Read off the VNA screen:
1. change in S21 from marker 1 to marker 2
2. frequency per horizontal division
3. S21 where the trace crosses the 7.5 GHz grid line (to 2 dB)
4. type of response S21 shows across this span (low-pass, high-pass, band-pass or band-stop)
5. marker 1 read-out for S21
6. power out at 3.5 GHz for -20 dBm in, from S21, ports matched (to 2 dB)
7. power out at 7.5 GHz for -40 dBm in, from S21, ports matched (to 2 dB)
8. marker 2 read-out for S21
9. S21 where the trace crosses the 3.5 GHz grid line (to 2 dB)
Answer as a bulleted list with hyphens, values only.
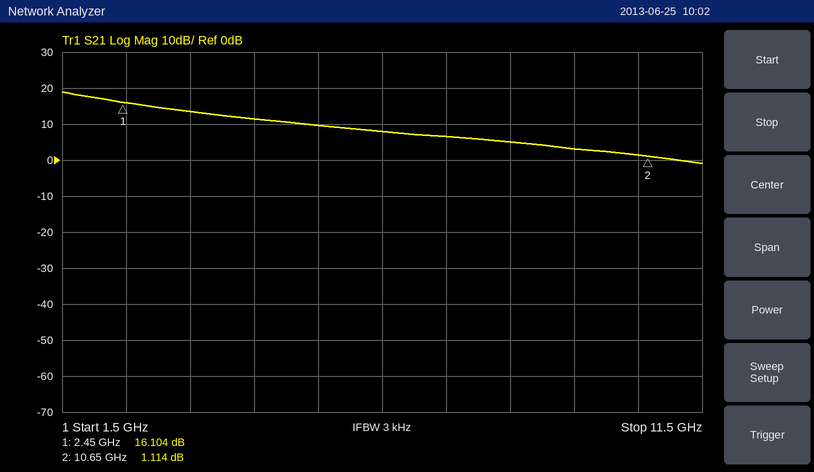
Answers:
- -14.990 dB
- 1 GHz
- 6 dB
- low-pass
- 16.104 dB
- -6 dBm
- -34 dBm
- 1.114 dB
- 14 dB
